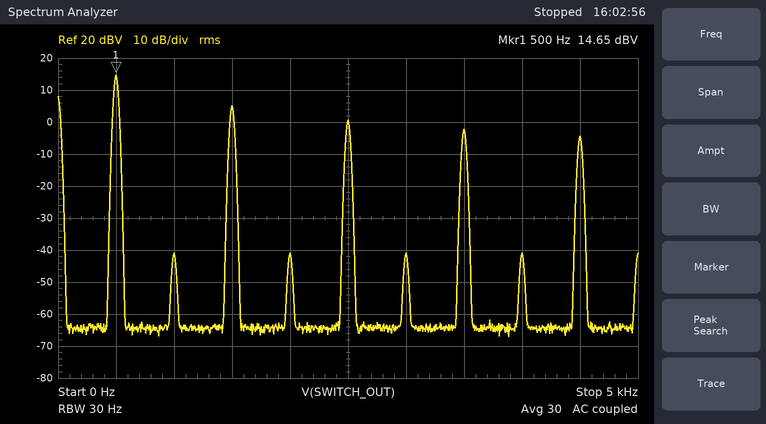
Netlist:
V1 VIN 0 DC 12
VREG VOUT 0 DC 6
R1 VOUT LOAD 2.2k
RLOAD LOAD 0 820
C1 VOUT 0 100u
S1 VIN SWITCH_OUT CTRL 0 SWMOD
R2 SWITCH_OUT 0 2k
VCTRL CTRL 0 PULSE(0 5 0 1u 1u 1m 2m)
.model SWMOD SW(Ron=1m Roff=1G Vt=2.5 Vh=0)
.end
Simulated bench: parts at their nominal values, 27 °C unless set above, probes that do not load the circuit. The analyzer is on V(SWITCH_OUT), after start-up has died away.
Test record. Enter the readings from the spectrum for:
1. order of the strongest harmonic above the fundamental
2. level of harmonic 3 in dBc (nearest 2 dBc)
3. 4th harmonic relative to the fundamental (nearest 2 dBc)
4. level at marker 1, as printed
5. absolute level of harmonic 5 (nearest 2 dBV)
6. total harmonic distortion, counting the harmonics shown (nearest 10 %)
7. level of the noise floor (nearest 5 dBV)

3
-10 dBc
-56 dBc
14.65 dBV
0 dBV
40 %
-65 dBV
